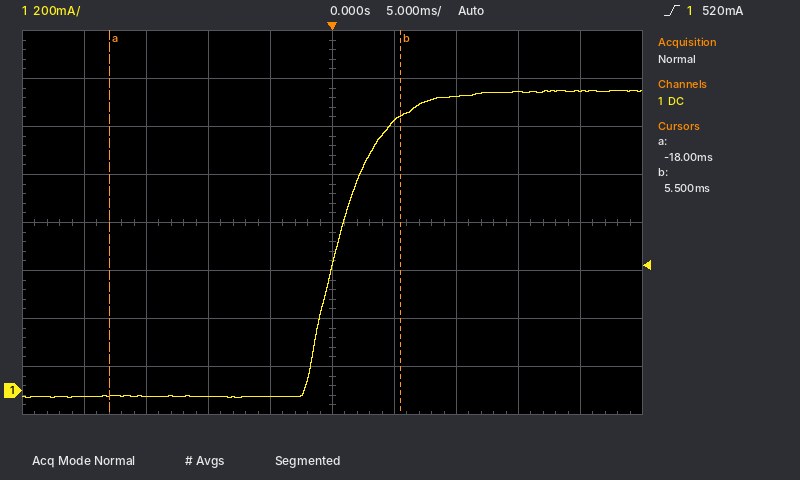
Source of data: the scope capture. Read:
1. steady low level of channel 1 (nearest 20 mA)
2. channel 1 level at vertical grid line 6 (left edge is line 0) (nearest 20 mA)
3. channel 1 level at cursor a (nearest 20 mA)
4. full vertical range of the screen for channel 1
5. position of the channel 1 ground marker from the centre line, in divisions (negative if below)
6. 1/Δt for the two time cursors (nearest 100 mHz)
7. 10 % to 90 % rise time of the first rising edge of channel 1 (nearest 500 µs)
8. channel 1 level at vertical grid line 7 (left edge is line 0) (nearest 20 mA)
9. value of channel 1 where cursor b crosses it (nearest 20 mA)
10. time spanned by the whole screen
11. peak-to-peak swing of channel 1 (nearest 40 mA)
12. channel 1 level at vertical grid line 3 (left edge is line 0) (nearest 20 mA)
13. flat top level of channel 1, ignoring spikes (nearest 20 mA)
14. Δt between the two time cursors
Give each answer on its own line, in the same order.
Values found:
-20 mA
1.12 A
-20 mA
1.6 A
-3.5 div
42.6 Hz
6.5 ms
1.22 A
1.14 A
50 ms
1.28 A
-20 mA
1.24 A
23.5 ms
